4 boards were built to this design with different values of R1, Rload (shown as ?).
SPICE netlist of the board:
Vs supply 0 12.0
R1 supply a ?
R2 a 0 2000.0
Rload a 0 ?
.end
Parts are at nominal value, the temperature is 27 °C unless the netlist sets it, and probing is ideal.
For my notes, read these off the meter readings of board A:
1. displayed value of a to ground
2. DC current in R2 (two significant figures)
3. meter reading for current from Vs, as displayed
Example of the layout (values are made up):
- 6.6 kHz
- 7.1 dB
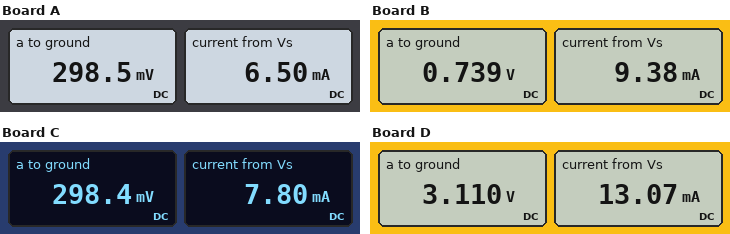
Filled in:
- 298.5 mV
- 150 µA
- 6.50 mA
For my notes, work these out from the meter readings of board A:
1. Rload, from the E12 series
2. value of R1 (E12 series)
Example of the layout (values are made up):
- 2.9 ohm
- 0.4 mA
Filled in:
- 47 Ω
- 1.8 kΩ
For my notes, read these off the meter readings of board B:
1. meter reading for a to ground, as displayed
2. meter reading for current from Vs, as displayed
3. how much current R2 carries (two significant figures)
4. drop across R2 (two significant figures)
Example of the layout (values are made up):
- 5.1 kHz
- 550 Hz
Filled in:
- 0.739 V
- 9.38 mA
- 370 µA
- 740 mV
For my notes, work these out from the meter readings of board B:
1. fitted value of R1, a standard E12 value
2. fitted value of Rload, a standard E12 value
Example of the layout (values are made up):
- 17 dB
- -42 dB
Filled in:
- 1.2 kΩ
- 82 Ω
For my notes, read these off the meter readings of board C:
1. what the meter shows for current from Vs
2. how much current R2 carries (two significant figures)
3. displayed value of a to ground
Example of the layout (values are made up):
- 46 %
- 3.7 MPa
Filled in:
- 7.80 mA
- 150 µA
- 298.4 mV
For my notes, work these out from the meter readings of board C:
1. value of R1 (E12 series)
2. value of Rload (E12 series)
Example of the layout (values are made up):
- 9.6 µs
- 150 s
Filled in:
- 1.5 kΩ
- 39 Ω
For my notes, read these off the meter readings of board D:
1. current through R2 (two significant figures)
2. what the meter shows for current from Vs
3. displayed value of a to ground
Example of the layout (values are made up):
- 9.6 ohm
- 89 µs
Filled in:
- 1.6 mA
- 13.07 mA
- 3.110 V
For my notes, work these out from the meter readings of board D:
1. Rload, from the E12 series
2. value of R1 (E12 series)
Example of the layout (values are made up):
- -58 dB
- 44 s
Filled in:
- 270 Ω
- 680 Ω
